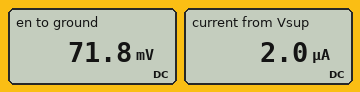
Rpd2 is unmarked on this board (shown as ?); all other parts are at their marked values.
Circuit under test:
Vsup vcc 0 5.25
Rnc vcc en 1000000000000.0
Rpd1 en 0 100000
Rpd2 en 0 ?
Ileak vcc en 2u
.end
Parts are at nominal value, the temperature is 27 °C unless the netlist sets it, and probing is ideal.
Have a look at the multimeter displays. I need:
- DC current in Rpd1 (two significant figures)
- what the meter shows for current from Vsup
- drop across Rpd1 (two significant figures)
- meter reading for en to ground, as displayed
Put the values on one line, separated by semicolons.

720 nA; 2.0 µA; 72 mV; 71.8 mV
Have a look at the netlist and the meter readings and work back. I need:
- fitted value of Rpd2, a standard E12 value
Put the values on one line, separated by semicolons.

56 kΩ
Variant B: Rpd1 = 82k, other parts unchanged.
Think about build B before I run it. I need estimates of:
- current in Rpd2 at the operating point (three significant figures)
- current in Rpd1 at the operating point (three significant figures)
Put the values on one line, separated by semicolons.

1.19 µA; 812 nA
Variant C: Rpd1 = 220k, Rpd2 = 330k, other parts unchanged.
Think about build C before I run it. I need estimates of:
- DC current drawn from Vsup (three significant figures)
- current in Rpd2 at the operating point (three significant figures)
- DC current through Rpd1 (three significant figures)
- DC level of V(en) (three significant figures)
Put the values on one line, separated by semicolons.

2.00 µA; 800 nA; 1.20 µA; 264 mV
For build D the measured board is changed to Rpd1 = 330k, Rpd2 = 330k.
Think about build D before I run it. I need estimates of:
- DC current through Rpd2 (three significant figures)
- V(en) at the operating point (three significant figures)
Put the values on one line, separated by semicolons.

1.00 µA; 330 mV
